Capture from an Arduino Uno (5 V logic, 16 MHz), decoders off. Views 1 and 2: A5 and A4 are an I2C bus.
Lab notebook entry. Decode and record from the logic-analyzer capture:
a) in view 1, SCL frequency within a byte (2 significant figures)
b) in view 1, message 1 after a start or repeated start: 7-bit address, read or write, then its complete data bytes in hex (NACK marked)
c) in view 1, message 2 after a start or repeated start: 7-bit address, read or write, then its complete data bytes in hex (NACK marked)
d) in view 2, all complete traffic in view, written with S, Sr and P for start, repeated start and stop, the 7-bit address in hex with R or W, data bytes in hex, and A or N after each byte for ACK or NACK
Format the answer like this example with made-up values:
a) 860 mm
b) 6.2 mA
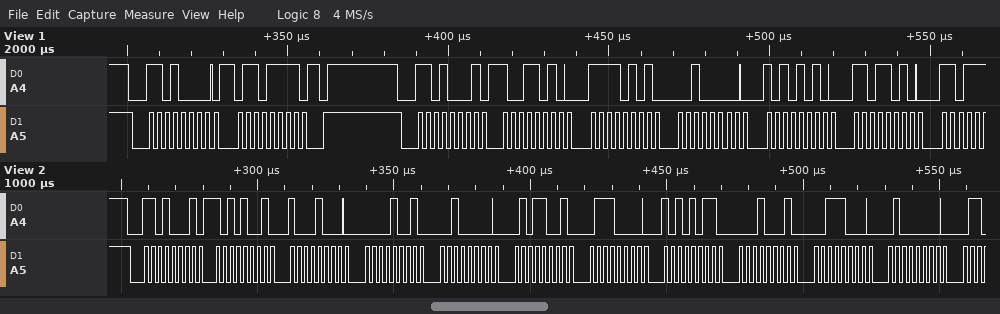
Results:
a) 400 kHz
b) 0x68 write: 6F
c) 0x68 read: 9A F5 20 AA DA
d) S 68R A A9 A 88 A 09 A 20 A 59 A 70 A AB A 11 A 38 A 40 A
